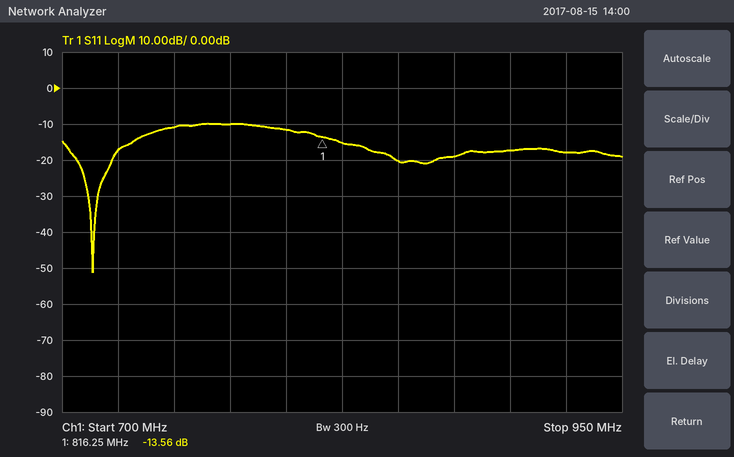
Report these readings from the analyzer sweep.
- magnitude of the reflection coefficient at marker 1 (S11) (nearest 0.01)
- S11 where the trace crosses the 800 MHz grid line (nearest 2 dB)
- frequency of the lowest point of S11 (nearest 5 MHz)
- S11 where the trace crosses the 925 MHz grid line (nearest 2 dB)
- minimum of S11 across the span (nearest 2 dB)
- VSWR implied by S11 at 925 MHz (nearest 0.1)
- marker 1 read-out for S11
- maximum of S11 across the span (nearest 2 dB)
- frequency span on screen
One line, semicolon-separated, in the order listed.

0.21; -12 dB; 715 MHz; -18 dB; -52 dB; 1.3; -13.56 dB; -10 dB; 250 MHz
